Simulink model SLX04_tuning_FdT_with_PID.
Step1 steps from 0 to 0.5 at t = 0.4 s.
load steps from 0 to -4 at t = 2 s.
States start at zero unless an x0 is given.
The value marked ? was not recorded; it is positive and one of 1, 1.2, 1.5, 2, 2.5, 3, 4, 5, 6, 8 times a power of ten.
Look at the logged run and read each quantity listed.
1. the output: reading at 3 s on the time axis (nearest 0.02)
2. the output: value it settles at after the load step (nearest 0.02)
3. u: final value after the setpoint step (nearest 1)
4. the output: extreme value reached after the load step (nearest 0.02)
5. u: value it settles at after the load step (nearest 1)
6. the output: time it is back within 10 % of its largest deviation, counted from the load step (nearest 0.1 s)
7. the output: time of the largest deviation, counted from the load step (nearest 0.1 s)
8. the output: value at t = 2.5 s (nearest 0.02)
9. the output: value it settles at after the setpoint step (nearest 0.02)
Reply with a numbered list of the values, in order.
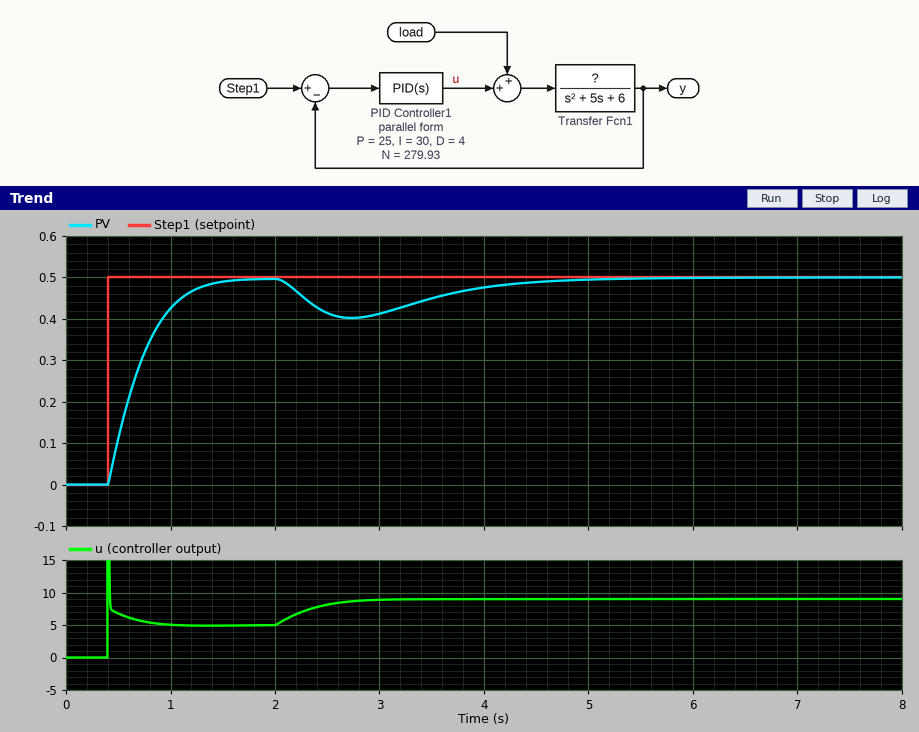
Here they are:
1. 0.42
2. 0.50
3. 5
4. 0.40
5. 9
6. 2.6 s
7. 0.7 s
8. 0.42
9. 0.50
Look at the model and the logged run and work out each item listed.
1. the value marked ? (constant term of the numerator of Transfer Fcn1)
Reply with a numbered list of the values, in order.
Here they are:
1. 0.6
